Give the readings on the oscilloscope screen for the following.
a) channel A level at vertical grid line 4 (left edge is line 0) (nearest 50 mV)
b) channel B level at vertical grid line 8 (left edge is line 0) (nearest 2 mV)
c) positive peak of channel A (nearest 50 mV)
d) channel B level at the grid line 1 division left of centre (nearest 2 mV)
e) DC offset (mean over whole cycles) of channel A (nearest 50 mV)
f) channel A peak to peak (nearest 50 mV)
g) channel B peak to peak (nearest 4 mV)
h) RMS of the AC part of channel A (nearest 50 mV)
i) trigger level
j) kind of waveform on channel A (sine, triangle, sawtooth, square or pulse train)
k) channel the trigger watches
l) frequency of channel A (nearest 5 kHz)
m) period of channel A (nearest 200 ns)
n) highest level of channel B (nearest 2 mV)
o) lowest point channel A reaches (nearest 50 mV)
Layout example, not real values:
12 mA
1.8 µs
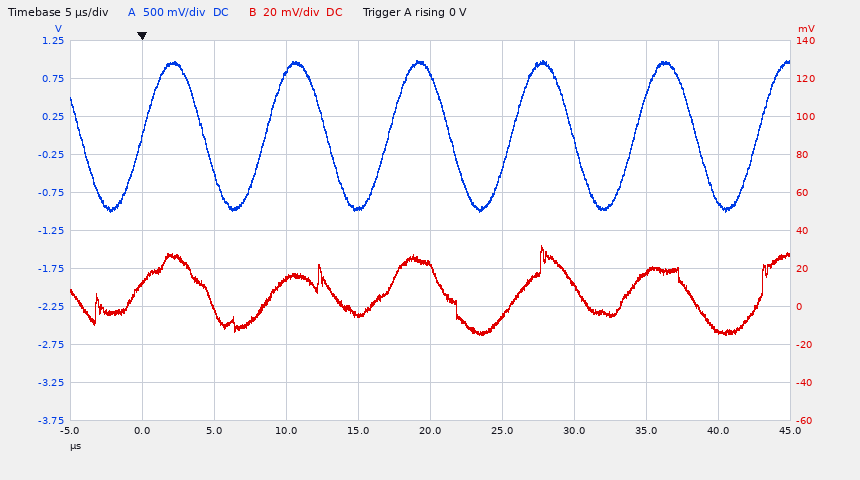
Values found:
-950 mV
18 mV
1.00 V
-4 mV
0 mV
2.00 V
48 mV
700 mV
0 V
sine
channel A
115 kHz
8.6 µs
32 mV
-1.00 V
